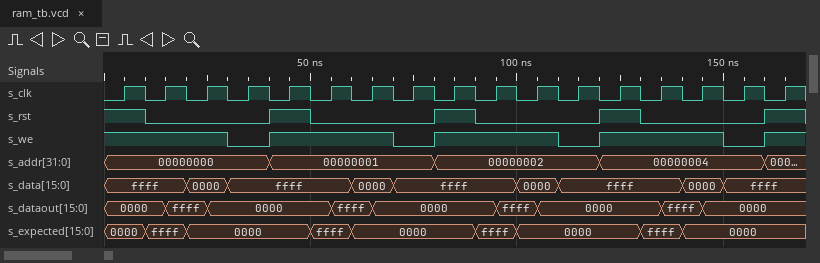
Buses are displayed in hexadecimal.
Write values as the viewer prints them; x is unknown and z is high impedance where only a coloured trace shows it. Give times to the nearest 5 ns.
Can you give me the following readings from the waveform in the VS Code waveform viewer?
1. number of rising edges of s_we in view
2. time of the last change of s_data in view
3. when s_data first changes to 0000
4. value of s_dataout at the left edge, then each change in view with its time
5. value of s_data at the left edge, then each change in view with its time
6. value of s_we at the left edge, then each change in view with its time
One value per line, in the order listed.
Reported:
4
150 ns
20 ns
0000, ffff at 15 ns, 0000 at 25 ns, ffff at 55 ns, 0000 at 65 ns, ffff at 95 ns, 0000 at 105 ns, ffff at 135 ns, 0000 at 145 ns
ffff, 0000 at 20 ns, ffff at 30 ns, 0000 at 60 ns, ffff at 70 ns, 0000 at 100 ns, ffff at 110 ns, 0000 at 140 ns, ffff at 150 ns
1, 0 at 30 ns, 1 at 40 ns, 0 at 70 ns, 1 at 80 ns, 0 at 110 ns, 1 at 120 ns, 0 at 150 ns, 1 at 160 ns
